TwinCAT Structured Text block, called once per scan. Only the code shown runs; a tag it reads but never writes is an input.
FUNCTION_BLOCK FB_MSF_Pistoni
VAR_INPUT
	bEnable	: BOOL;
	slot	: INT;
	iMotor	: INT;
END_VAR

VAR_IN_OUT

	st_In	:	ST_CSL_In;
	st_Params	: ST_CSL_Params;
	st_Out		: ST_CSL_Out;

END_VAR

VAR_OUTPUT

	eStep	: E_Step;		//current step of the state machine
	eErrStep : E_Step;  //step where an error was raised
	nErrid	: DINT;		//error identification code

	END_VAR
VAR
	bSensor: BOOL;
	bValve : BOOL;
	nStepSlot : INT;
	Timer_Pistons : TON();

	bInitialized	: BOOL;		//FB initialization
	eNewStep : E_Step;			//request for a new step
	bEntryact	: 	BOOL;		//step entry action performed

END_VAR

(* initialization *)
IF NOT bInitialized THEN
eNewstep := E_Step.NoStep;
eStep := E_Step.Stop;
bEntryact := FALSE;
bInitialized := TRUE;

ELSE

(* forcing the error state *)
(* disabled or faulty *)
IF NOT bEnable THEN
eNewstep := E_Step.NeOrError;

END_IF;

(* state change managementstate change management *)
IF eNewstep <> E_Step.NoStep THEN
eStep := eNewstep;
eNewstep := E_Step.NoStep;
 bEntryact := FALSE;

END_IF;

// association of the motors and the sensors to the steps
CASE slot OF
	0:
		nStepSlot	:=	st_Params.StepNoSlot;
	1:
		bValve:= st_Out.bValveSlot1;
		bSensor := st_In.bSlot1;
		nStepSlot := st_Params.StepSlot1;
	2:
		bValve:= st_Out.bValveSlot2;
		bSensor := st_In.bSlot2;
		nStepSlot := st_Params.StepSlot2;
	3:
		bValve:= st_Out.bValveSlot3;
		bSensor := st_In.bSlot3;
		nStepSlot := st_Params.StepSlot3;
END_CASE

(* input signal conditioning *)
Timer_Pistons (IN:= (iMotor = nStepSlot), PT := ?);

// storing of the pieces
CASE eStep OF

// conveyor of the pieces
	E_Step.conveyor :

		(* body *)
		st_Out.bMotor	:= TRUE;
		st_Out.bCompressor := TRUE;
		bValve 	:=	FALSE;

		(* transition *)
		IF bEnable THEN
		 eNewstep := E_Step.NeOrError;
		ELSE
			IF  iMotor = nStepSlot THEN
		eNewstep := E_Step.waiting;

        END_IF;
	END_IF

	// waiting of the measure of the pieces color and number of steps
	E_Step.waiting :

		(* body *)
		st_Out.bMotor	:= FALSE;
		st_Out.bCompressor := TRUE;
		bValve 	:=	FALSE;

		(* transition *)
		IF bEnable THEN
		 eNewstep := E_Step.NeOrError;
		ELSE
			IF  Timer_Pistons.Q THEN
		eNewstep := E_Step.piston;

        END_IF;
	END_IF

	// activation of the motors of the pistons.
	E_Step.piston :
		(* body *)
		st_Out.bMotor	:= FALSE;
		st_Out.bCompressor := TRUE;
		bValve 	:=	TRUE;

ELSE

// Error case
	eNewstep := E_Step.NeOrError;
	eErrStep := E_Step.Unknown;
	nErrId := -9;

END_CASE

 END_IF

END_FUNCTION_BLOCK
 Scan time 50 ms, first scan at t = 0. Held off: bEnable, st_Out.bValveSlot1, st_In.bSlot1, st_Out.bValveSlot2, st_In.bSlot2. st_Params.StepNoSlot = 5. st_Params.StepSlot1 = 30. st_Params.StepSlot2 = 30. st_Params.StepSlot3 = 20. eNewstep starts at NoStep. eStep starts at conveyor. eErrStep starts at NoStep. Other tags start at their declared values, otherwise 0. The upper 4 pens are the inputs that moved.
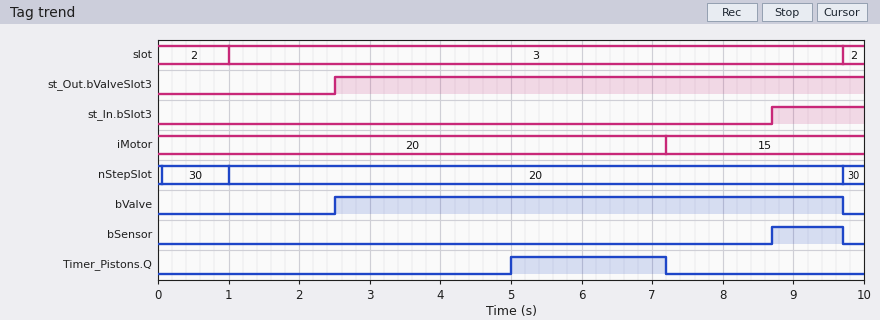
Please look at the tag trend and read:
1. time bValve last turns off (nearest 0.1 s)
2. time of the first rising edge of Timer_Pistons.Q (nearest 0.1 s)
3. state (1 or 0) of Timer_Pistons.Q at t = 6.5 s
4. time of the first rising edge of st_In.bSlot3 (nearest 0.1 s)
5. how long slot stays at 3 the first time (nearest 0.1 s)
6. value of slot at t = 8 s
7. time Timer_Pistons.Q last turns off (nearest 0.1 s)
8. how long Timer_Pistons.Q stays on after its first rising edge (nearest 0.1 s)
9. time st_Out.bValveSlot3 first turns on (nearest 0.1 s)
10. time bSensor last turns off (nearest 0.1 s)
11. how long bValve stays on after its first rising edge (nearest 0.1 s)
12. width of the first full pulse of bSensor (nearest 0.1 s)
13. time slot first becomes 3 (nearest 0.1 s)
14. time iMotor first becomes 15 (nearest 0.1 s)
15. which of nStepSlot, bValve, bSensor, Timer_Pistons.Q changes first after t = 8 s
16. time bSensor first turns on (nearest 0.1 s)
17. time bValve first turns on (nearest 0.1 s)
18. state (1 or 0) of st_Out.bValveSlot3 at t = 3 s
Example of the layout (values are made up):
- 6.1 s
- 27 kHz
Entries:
- 9.7 s
- 5.0 s
- 1
- 8.7 s
- 8.7 s
- 3
- 7.2 s
- 2.2 s
- 2.5 s
- 9.7 s
- 7.2 s
- 1.0 s
- 1.0 s
- 7.2 s
- bSensor
- 8.7 s
- 2.5 s
- 1
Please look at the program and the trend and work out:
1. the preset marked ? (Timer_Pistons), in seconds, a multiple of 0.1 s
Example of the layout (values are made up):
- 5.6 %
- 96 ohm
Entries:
- 4.0 s
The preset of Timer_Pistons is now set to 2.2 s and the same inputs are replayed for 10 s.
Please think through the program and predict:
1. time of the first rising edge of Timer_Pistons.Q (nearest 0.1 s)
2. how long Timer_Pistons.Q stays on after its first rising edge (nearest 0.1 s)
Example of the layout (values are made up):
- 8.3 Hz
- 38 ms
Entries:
- 3.2 s
- 4.0 s
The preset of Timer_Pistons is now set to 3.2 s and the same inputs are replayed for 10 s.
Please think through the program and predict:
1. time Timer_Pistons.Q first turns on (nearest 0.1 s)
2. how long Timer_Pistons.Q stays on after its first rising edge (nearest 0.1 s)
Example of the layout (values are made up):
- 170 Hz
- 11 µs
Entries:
- 4.2 s
- 3.0 s
